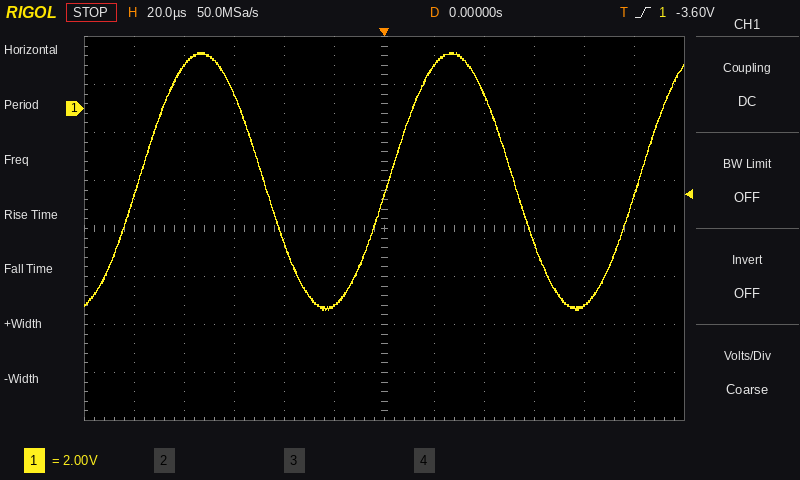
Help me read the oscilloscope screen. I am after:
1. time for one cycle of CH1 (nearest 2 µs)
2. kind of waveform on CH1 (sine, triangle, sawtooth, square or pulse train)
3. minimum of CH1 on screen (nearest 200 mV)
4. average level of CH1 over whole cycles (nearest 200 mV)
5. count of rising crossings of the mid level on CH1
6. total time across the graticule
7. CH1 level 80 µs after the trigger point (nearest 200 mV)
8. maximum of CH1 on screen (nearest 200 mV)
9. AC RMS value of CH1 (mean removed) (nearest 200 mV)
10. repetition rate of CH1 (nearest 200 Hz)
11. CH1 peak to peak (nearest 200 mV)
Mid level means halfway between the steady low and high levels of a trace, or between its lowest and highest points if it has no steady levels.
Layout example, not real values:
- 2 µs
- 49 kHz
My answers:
- 100 µs
- sine
- -8.4 V
- -3.0 V
- 3
- 240 µs
- -8.2 V
- 2.4 V
- 3.8 V
- 10.0 kHz
- 10.8 V
